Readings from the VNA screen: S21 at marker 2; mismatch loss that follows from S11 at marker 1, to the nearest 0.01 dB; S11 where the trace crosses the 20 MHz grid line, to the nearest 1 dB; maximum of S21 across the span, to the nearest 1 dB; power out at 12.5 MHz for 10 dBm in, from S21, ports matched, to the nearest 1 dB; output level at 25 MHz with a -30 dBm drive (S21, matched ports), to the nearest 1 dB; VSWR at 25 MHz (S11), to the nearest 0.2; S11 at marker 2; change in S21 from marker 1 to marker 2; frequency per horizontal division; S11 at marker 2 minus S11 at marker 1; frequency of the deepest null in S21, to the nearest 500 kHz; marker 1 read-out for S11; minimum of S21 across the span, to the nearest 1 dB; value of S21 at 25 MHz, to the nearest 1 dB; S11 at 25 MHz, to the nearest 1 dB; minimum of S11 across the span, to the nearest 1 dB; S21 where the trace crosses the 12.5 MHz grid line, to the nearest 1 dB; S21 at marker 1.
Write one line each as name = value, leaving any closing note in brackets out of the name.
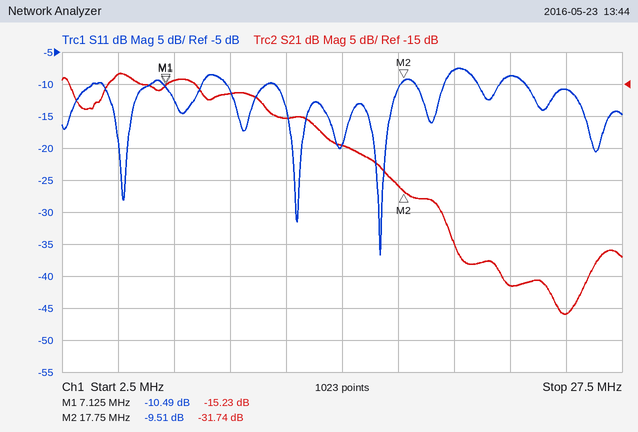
S21 at marker 2 = -31.74 dB
mismatch loss that follows from S11 at marker 1, to the nearest 0.01 dB = 0.41 dB
S11 where the trace crosses the 20 MHz grid line, to the nearest 1 dB = -8 dB
maximum of S21 across the span, to the nearest 1 dB = -13 dB
power out at 12.5 MHz for 10 dBm in, from S21, ports matched, to the nearest 1 dB = -10 dBm
output level at 25 MHz with a -30 dBm drive (S21, matched ports), to the nearest 1 dB = -81 dBm
VSWR at 25 MHz (S11), to the nearest 0.2 = 1.8
S11 at marker 2 = -9.51 dB
change in S21 from marker 1 to marker 2 = -16.51 dB
frequency per horizontal division = 2.5 MHz
S11 at marker 2 minus S11 at marker 1 = 0.98 dB
frequency of the deepest null in S21, to the nearest 500 kHz = 25.0 MHz
marker 1 read-out for S11 = -10.49 dB
minimum of S21 across the span, to the nearest 1 dB = -51 dB
value of S21 at 25 MHz, to the nearest 1 dB = -51 dB
S11 at 25 MHz, to the nearest 1 dB = -11 dB
minimum of S11 across the span, to the nearest 1 dB = -37 dB
S21 where the trace crosses the 12.5 MHz grid line, to the nearest 1 dB = -20 dB
S21 at marker 1 = -15.23 dB
